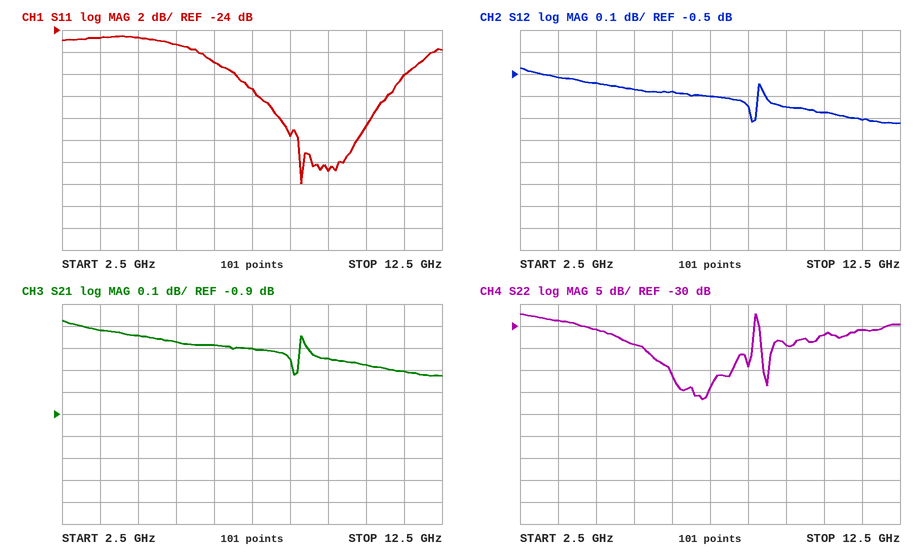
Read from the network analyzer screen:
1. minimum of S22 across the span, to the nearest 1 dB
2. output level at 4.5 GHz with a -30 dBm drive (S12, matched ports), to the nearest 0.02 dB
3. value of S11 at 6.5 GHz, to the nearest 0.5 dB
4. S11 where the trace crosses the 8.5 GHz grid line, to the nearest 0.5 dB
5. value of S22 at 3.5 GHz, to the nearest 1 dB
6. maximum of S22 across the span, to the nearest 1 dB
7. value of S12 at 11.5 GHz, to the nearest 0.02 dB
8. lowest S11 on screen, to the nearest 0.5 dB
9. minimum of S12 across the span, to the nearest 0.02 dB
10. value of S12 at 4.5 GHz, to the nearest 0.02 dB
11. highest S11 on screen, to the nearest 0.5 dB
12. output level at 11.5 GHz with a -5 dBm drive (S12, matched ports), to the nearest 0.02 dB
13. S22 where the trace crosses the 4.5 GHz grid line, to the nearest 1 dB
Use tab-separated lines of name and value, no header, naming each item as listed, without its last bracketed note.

minimum of S22 across the span, to the nearest 1 dB	-47 dB
output level at 4.5 GHz with a -30 dBm drive (S12, matched ports), to the nearest 0.02 dB	-30.54 dBm
value of S11 at 6.5 GHz, to the nearest 0.5 dB	-27.0 dB
S11 where the trace crosses the 8.5 GHz grid line, to the nearest 0.5 dB	-33.5 dB
value of S22 at 3.5 GHz, to the nearest 1 dB	-29 dB
maximum of S22 across the span, to the nearest 1 dB	-27 dB
value of S12 at 11.5 GHz, to the nearest 0.02 dB	-0.70 dB
lowest S11 on screen, to the nearest 0.5 dB	-38.0 dB
minimum of S12 across the span, to the nearest 0.02 dB	-0.72 dB
value of S12 at 4.5 GHz, to the nearest 0.02 dB	-0.54 dB
highest S11 on screen, to the nearest 0.5 dB	-24.5 dB
output level at 11.5 GHz with a -5 dBm drive (S12, matched ports), to the nearest 0.02 dB	-5.70 dBm
S22 where the trace crosses the 4.5 GHz grid line, to the nearest 1 dB	-31 dB
